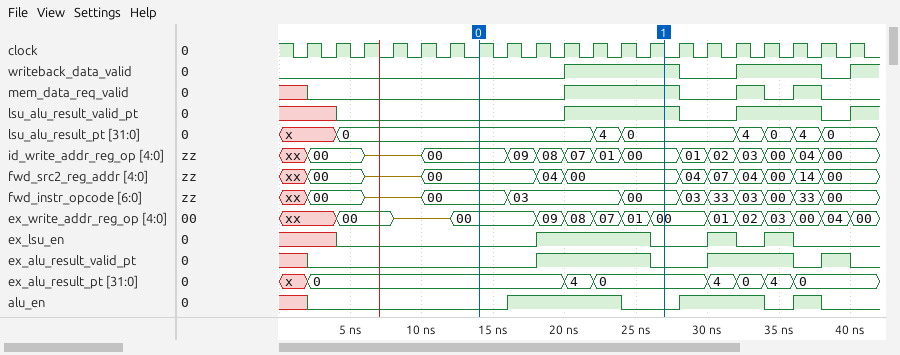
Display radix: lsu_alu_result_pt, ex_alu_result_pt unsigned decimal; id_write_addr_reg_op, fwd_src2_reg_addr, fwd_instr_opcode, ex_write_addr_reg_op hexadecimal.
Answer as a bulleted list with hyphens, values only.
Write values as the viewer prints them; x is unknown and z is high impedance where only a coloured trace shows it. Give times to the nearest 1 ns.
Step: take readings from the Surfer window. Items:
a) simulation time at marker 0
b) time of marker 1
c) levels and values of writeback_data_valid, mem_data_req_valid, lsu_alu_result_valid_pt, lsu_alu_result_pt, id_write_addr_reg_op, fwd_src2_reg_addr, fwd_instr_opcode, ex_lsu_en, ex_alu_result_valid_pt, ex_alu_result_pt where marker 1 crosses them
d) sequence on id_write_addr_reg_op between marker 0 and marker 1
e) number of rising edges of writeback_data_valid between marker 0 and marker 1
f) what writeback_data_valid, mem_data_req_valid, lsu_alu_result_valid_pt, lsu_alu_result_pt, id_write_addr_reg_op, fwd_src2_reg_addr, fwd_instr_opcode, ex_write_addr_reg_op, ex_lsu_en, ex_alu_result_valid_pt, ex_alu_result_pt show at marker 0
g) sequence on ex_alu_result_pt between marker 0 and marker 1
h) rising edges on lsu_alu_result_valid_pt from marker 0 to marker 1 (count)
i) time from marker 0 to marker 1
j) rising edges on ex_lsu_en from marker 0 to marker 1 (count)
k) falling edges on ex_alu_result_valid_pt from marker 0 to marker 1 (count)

- 14 ns
- 27 ns
- writeback_data_valid=1, mem_data_req_valid=1, lsu_alu_result_valid_pt=1, lsu_alu_result_pt=0, id_write_addr_reg_op=00, fwd_src2_reg_addr=00, fwd_instr_opcode=00, ex_lsu_en=0, ex_alu_result_valid_pt=0, ex_alu_result_pt=0
- 00, 09, 08, 07, 01, 00
- 1
- writeback_data_valid=0, mem_data_req_valid=0, lsu_alu_result_valid_pt=0, lsu_alu_result_pt=0, id_write_addr_reg_op=00, fwd_src2_reg_addr=00, fwd_instr_opcode=00, ex_write_addr_reg_op=00, ex_lsu_en=0, ex_alu_result_valid_pt=0, ex_alu_result_pt=0
- 0, 4, 0
- 1
- 13 ns
- 1
- 1
